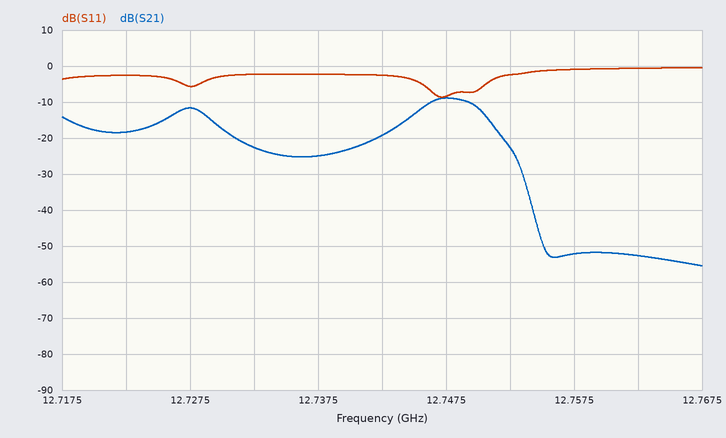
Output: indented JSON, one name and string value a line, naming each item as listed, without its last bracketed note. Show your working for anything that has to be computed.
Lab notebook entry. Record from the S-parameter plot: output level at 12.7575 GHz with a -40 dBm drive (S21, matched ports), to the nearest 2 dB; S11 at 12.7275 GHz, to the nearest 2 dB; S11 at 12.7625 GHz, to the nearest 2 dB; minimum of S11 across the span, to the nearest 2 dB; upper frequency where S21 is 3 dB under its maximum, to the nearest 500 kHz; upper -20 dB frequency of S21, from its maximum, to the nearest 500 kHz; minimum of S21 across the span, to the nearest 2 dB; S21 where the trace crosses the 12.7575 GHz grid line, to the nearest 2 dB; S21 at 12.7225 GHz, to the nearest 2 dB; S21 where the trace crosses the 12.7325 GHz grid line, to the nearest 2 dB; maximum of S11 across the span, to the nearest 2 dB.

{
  "output level at 12.7575 GHz with a -40 dBm drive (S21, matched ports), to the nearest 2 dB": "-40 dBm + (-52 dB) = -92 dBm",
  "S11 at 12.7275 GHz, to the nearest 2 dB": "-6 dB",
  "S11 at 12.7625 GHz, to the nearest 2 dB": "0 dB",
  "minimum of S11 across the span, to the nearest 2 dB": "-8 dB",
  "upper frequency where S21 is 3 dB under its maximum, to the nearest 500 kHz": "12.7500 GHz",
  "upper -20 dB frequency of S21, from its maximum, to the nearest 500 kHz": "12.7535 GHz",
  "minimum of S21 across the span, to the nearest 2 dB": "-56 dB",
  "S21 where the trace crosses the 12.7575 GHz grid line, to the nearest 2 dB": "-52 dB",
  "S21 at 12.7225 GHz, to the nearest 2 dB": "-18 dB",
  "S21 where the trace crosses the 12.7325 GHz grid line, to the nearest 2 dB": "-22 dB",
  "maximum of S11 across the span, to the nearest 2 dB": "0 dB"
}
